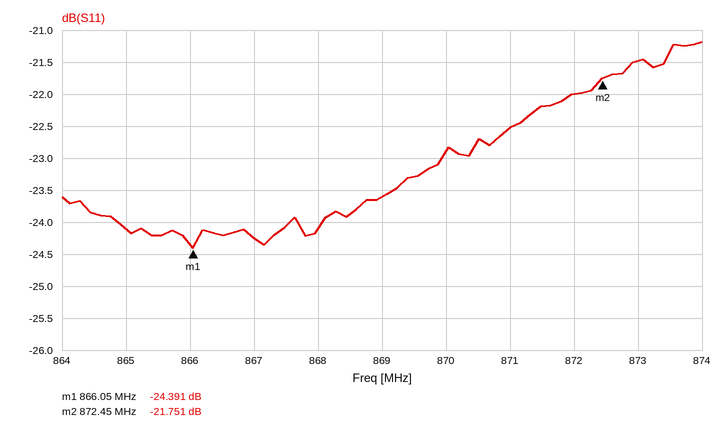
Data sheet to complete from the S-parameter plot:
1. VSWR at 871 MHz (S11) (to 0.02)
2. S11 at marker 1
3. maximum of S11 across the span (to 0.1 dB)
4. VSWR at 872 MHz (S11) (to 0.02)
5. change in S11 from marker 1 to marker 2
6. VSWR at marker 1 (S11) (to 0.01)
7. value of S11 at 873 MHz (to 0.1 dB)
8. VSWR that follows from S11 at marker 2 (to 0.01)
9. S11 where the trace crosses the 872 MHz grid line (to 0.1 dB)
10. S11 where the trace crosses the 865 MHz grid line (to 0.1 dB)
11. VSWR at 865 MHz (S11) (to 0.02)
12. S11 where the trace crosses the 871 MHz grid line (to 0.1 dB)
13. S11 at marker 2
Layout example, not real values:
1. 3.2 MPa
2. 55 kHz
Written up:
1. 1.16
2. -24.391 dB
3. -21.2 dB
4. 1.18
5. 2.640 dB
6. 1.13
7. -21.5 dB
8. 1.18
9. -22.0 dB
10. -24.1 dB
11. 1.14
12. -22.5 dB
13. -21.751 dB
